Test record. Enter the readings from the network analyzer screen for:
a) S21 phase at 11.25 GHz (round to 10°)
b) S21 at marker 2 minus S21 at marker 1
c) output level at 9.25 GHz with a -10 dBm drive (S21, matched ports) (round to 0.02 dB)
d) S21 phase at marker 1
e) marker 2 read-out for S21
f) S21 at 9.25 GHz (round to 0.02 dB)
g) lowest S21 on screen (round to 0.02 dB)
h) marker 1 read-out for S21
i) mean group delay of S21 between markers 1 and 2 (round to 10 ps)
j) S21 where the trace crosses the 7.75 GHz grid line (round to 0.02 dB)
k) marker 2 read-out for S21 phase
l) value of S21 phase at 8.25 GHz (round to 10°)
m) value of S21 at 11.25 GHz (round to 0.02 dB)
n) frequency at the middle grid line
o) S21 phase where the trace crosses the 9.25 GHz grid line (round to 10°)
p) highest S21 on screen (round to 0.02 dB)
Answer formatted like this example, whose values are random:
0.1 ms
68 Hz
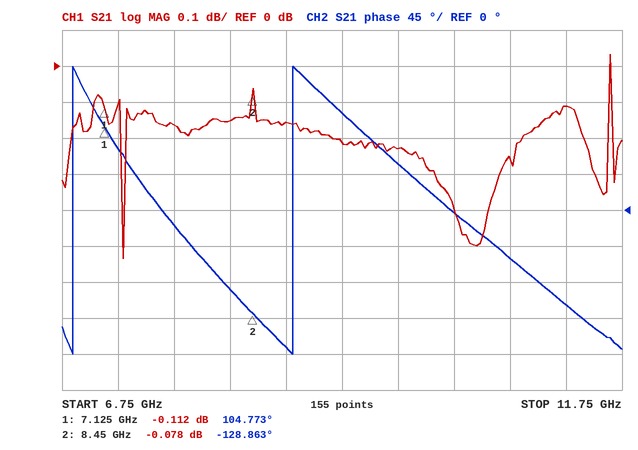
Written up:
-120°
0.034 dB
-10.22 dBm
104.773°
-0.078 dB
-0.22 dB
-0.54 dB
-0.112 dB
490 ps
-0.16 dB
-128.863°
-100°
-0.12 dB
9.25 GHz
120°
0.04 dB
